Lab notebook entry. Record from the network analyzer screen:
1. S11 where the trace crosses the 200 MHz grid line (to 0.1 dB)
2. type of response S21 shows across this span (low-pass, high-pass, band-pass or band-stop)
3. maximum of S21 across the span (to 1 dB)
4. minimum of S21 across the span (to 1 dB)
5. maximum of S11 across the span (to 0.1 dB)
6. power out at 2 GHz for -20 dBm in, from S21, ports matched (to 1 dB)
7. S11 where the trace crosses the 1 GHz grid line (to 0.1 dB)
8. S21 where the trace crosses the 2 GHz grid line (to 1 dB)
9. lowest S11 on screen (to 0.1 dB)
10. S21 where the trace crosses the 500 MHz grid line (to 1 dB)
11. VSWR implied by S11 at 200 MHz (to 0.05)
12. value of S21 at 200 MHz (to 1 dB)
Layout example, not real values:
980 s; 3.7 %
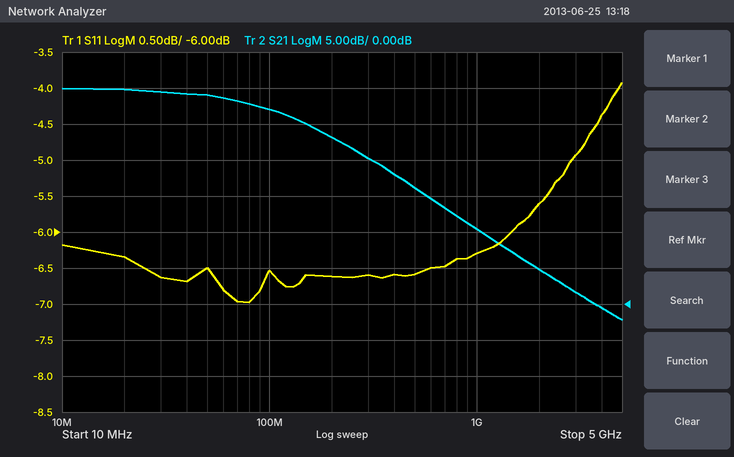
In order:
-6.6 dB; low-pass; 30 dB; -2 dB; -3.9 dB; -15 dBm; -6.3 dB; 5 dB; -7.0 dB; 16 dB; 2.75; 23 dB
